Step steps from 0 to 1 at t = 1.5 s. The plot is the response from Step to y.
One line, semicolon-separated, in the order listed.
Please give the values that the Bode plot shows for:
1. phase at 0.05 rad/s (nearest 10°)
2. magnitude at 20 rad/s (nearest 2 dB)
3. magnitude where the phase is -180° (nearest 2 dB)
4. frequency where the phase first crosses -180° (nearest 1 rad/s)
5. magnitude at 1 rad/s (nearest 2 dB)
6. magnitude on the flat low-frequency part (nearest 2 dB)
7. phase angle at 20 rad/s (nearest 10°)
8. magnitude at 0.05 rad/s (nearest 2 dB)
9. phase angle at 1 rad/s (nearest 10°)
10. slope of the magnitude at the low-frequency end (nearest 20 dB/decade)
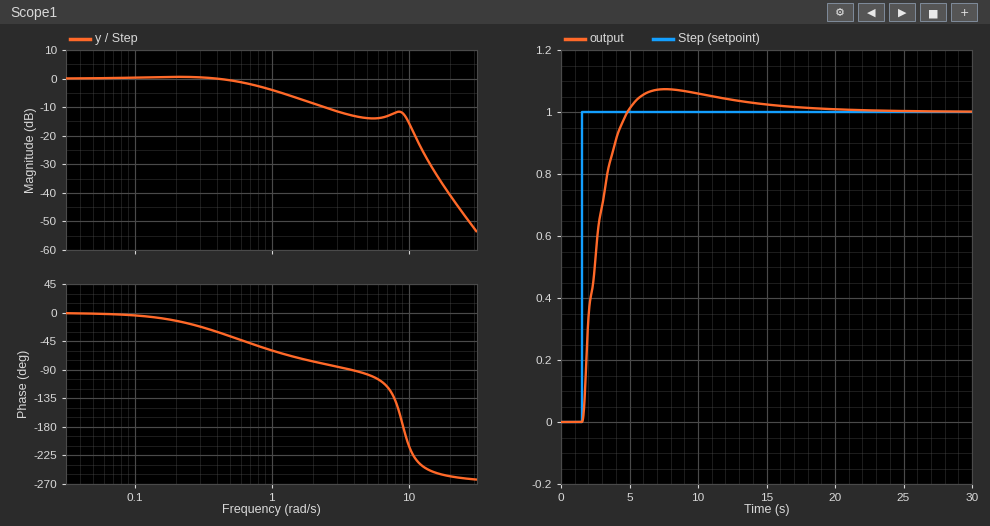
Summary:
0°; -40 dB; -12 dB; 9 rad/s; -4 dB; 0 dB; -260°; 0 dB; -60°; 0 dB/decade
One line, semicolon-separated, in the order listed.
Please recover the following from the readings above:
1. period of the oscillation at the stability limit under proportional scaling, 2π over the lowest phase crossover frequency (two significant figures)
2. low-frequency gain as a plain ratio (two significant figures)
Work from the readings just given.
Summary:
0.70 s; 1.0
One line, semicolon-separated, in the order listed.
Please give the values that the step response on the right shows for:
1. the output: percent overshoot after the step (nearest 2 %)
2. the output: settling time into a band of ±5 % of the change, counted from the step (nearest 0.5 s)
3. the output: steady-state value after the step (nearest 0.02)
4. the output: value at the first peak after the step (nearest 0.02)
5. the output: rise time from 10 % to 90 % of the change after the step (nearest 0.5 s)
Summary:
8 %; 9.5 s; 1.00; 1.08; 2.0 s
